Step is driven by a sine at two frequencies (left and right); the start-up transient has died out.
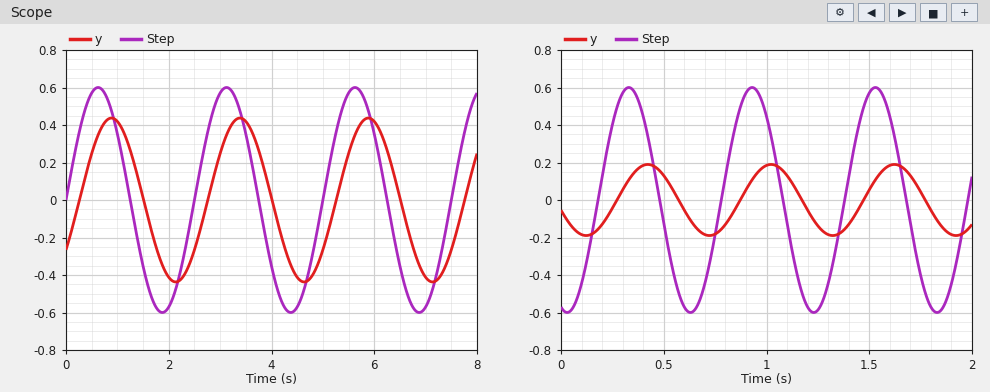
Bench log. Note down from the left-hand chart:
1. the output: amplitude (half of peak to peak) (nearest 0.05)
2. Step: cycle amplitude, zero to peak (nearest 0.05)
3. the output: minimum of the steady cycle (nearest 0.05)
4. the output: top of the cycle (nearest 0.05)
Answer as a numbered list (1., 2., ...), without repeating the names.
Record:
1. 0.45
2. 0.60
3. -0.45
4. 0.45
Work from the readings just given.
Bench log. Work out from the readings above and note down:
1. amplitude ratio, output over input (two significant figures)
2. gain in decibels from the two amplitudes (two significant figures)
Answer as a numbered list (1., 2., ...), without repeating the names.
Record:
1. 0.75
2. -2.5 dB
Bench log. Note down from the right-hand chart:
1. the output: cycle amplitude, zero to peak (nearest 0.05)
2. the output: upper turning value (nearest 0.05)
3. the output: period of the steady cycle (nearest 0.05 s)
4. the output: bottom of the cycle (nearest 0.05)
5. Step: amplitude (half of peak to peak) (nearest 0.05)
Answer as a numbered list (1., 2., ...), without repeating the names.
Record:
1. 0.20
2. 0.20
3. 0.60 s
4. -0.20
5. 0.60
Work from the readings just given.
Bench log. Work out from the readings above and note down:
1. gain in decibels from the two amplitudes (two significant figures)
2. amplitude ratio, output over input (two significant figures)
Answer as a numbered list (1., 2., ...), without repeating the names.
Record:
1. -9.5 dB
2. 0.33
